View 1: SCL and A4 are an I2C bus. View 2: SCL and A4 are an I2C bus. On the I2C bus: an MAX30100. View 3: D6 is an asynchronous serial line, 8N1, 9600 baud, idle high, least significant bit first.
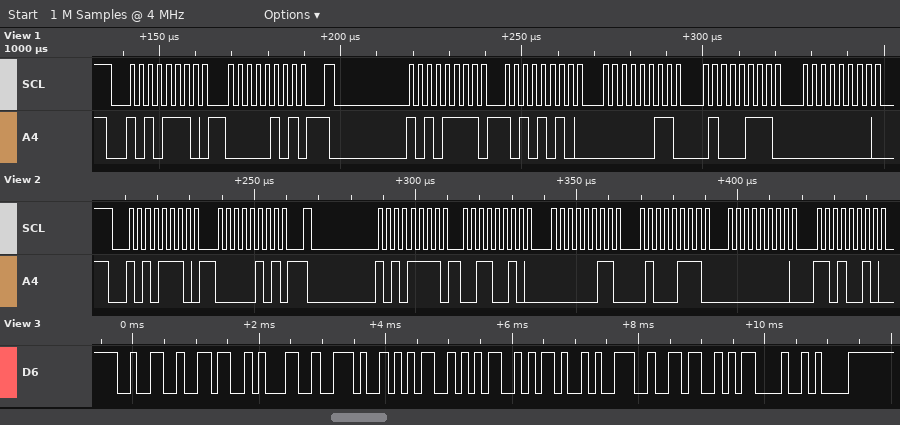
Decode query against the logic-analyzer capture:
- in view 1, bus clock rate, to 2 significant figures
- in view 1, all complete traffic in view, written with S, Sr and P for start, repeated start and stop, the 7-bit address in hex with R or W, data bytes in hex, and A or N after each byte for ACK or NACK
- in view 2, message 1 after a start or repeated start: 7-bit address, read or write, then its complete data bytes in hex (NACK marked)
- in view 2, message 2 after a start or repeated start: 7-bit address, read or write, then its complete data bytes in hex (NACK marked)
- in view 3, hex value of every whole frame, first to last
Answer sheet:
400 kHz
S 57W A 05 A Sr 57R A AA A 03 A 47 A 00 A
0x57 write: 05
0x57 read: 32 03 47 00 D2
32 36 31 2E 35 35 2D 39 36 0D 0A
